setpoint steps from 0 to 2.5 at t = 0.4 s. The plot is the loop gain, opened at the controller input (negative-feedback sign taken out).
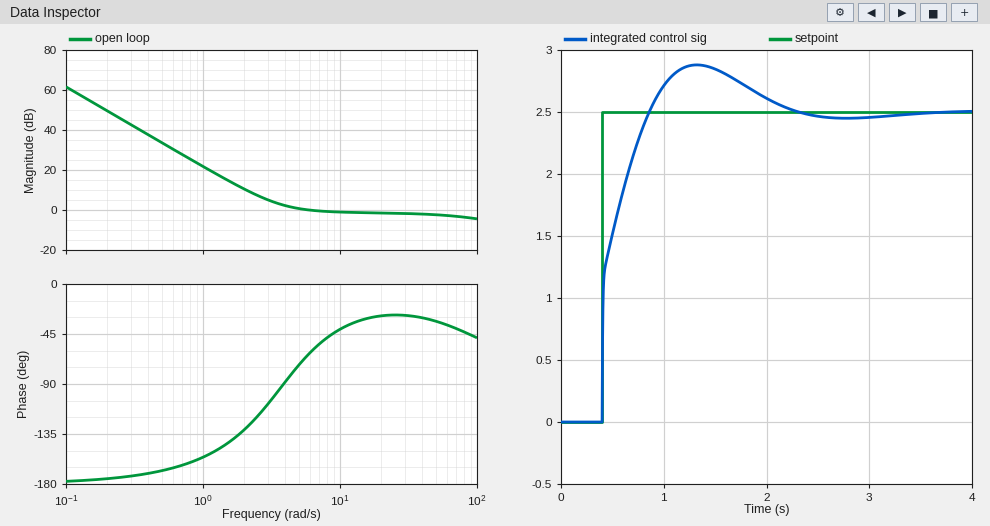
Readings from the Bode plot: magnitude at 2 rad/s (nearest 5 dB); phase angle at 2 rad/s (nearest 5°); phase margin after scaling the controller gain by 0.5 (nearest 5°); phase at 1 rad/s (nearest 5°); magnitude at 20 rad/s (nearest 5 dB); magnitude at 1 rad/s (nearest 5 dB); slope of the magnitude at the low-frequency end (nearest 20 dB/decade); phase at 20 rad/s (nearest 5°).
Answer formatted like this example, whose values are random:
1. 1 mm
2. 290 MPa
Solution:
1. 10 dB
2. -130°
3. 65°
4. -155°
5. 0 dB
6. 20 dB
7. -40 dB/decade
8. -30°
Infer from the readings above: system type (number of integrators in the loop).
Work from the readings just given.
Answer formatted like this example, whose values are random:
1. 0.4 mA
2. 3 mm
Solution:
1. 2
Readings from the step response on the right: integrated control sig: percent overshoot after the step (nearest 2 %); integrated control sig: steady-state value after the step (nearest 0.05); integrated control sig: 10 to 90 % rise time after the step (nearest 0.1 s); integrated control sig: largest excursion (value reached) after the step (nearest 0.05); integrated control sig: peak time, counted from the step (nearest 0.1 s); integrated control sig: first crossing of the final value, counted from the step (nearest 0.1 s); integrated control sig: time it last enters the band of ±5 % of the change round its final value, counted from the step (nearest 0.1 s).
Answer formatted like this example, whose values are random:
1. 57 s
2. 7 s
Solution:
1. 16 %
2. 2.50
3. 0.3 s
4. 2.90
5. 0.9 s
6. 0.5 s
7. 1.6 s
